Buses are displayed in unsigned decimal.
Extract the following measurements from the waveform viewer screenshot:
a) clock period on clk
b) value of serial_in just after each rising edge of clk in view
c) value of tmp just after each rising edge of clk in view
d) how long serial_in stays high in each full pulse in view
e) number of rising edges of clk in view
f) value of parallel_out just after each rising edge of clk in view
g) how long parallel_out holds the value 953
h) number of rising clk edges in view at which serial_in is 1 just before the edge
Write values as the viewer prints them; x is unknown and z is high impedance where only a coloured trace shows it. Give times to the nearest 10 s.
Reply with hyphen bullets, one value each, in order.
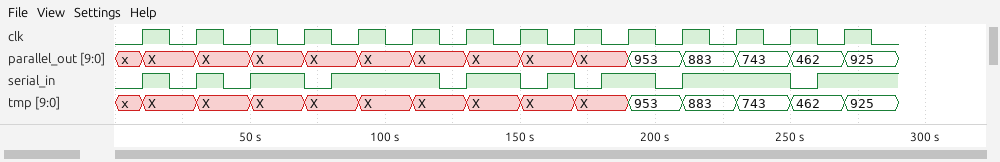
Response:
- 20 s
- 1 1 1 0 1 1 1 0 0 1 1 1 0 1
- X, X, X, X, X, X, X, X, X, 953, 883, 743, 462, 925
- 10 s, 10 s, 20 s, 40 s, 20 s, 10 s, 20 s, 40 s
- 14
- X, X, X, X, X, X, X, X, X, 953, 883, 743, 462, 925
- 20 s
- 9
